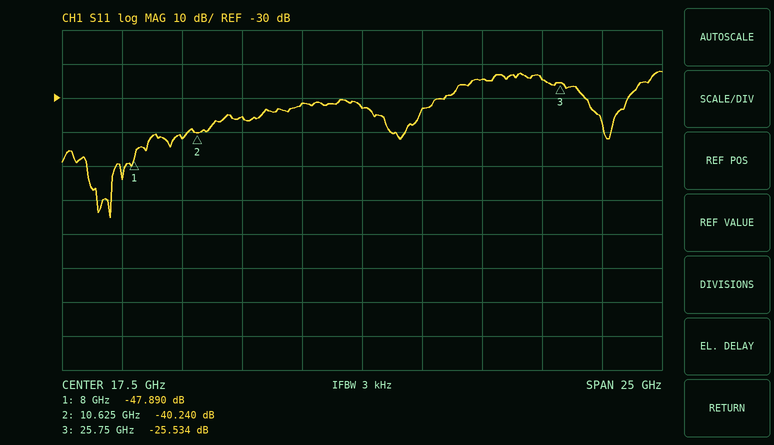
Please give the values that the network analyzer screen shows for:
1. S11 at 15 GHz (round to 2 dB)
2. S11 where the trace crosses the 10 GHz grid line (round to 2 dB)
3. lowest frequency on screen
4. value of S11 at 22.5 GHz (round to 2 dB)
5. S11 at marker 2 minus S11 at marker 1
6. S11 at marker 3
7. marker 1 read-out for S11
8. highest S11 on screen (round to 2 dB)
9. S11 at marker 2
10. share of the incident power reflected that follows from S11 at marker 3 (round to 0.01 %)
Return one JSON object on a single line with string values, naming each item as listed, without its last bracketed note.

{"S11 at 15 GHz": "-32 dB", "S11 where the trace crosses the 10 GHz grid line": "-42 dB", "lowest frequency on screen": "5 GHz", "value of S11 at 22.5 GHz": "-24 dB", "S11 at marker 2 minus S11 at marker 1": "7.650 dB", "S11 at marker 3": "-25.534 dB", "marker 1 read-out for S11": "-47.890 dB", "highest S11 on screen": "-22 dB", "S11 at marker 2": "-40.240 dB", "share of the incident power reflected that follows from S11 at marker 3": "0.28 %"}
